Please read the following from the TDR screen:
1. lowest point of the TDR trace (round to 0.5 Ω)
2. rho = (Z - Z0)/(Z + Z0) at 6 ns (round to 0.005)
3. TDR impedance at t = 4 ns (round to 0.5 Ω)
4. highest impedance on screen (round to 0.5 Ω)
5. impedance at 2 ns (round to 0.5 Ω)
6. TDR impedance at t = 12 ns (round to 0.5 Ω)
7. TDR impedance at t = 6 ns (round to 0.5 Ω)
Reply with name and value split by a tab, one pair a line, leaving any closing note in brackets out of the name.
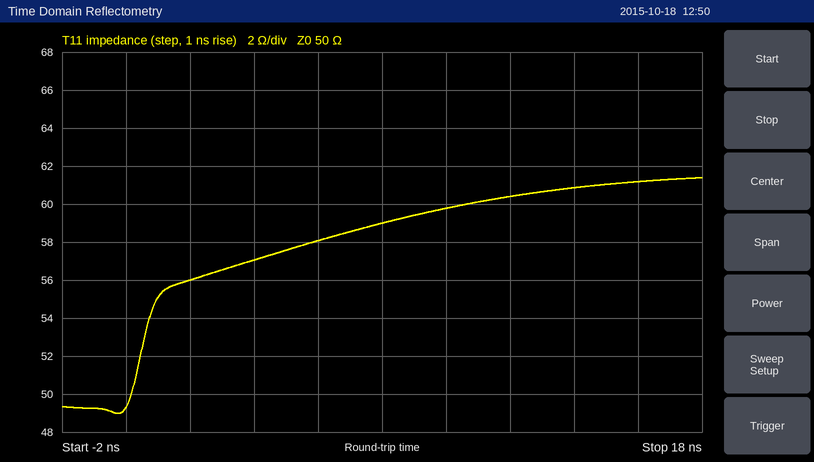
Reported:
lowest point of the TDR trace	49.0 Ω
rho = (Z - Z0)/(Z + Z0) at 6 ns	+0.075
TDR impedance at t = 4 ns	57.0 Ω
highest impedance on screen	61.5 Ω
impedance at 2 ns	56.0 Ω
TDR impedance at t = 12 ns	60.5 Ω
TDR impedance at t = 6 ns	58.0 Ω
